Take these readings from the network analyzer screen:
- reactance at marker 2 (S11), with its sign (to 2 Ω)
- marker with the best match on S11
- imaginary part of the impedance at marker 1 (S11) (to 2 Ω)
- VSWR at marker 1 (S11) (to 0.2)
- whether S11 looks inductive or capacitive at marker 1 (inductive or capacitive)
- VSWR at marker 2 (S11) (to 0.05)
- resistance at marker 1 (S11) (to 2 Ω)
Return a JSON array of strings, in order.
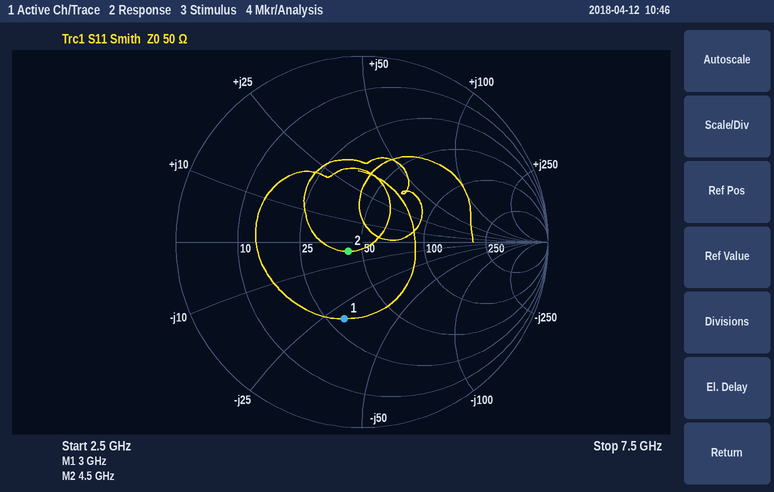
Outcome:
["-4 Ω", "marker 2", "-30 Ω", "2.4", "capacitive", "1.20", "30 Ω"]
